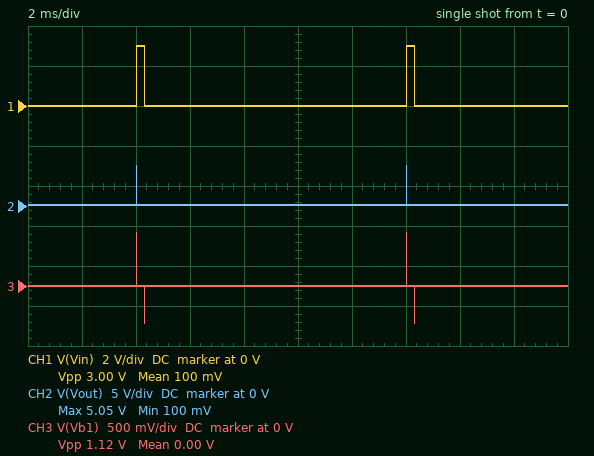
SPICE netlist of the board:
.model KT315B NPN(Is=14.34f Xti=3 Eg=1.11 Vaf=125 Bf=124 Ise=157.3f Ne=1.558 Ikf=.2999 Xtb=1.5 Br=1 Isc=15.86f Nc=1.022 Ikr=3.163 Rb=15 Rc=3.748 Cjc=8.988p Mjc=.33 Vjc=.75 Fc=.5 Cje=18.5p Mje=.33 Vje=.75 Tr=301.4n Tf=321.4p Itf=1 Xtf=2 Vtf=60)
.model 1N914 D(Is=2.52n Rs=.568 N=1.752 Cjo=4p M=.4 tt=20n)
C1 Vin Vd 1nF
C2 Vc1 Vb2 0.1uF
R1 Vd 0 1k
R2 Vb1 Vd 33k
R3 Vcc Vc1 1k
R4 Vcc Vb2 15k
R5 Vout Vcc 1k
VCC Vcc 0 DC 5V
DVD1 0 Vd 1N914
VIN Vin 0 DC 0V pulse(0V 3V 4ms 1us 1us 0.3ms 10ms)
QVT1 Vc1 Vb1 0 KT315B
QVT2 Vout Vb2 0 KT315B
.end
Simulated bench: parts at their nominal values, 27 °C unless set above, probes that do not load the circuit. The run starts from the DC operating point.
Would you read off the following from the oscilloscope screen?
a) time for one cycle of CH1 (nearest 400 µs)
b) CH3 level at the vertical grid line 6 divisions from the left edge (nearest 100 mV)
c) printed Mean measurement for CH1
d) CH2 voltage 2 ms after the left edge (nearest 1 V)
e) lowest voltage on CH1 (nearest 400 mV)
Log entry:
10.0 ms
0 V
100 mV
0 V
0 V
